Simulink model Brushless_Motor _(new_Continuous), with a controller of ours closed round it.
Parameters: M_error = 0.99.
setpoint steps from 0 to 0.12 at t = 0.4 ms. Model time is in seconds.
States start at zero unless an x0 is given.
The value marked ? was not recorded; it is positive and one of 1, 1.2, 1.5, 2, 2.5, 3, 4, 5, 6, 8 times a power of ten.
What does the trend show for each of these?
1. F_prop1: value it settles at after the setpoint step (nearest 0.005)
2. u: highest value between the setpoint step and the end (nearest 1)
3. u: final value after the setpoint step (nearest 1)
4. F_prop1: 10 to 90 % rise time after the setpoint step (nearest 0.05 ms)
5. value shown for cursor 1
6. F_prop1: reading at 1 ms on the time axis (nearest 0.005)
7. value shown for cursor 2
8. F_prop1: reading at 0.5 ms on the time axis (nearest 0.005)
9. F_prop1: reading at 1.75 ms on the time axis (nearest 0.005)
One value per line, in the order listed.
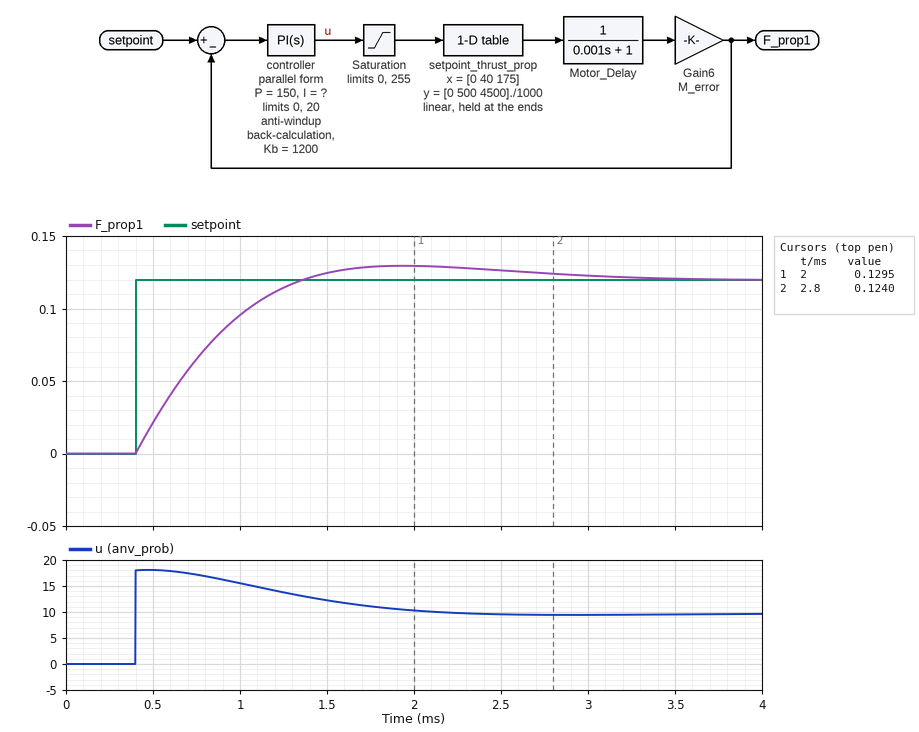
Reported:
0.120
18
10
0.70 ms
0.1295
0.095
0.1240
0.020
0.130
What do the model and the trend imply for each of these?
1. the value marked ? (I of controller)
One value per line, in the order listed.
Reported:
300000
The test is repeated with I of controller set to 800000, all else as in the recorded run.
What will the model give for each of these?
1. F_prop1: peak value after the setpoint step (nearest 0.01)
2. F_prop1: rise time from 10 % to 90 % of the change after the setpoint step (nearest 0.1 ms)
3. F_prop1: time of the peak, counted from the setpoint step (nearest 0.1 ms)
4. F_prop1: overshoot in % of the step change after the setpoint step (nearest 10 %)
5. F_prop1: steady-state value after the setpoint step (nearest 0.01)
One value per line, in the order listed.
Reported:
0.15
0.5 ms
1.1 ms
30 %
0.12
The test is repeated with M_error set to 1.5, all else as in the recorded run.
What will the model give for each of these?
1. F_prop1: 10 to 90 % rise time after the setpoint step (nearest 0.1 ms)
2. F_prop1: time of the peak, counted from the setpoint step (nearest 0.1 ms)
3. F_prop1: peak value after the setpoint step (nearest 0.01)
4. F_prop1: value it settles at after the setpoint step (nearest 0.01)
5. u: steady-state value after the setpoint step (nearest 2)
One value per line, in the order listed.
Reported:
0.5 ms
1.2 ms
0.13
0.12
6
